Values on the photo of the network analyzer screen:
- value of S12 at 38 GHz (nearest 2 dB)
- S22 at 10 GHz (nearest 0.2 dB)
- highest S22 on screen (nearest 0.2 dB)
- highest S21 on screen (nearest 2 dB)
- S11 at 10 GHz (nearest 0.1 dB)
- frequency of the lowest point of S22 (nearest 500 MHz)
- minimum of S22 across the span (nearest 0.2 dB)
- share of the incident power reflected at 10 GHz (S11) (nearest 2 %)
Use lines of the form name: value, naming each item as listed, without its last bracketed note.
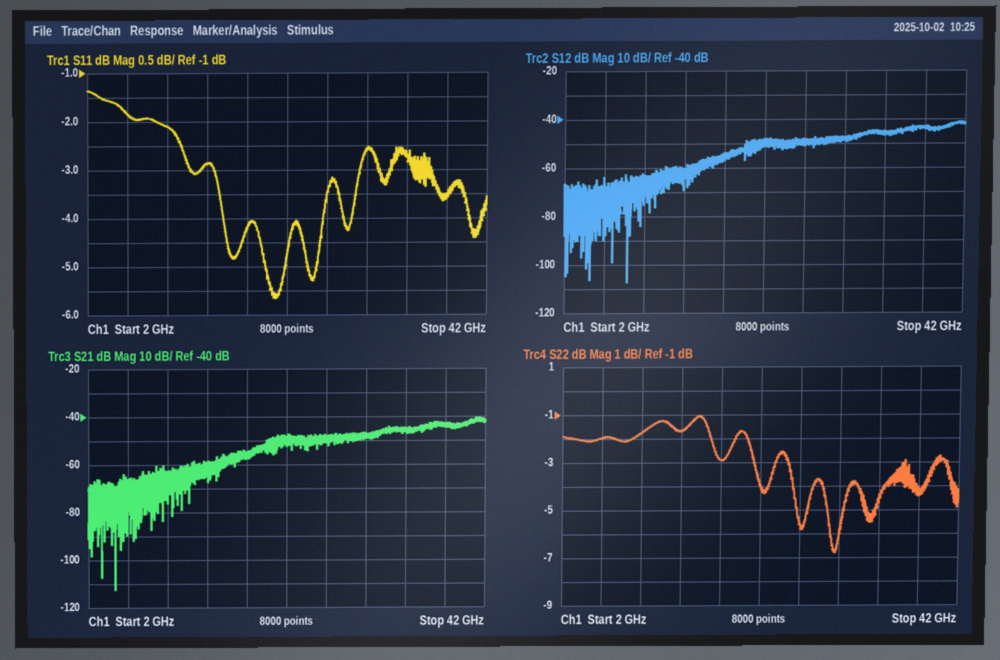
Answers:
value of S12 at 38 GHz: -44 dB
S22 at 10 GHz: -1.8 dB
highest S22 on screen: -1.0 dB
highest S21 on screen: -40 dB
S11 at 10 GHz: -2.1 dB
frequency of the lowest point of S22: 29.5 GHz
minimum of S22 across the span: -6.8 dB
share of the incident power reflected at 10 GHz (S11): 62 %
